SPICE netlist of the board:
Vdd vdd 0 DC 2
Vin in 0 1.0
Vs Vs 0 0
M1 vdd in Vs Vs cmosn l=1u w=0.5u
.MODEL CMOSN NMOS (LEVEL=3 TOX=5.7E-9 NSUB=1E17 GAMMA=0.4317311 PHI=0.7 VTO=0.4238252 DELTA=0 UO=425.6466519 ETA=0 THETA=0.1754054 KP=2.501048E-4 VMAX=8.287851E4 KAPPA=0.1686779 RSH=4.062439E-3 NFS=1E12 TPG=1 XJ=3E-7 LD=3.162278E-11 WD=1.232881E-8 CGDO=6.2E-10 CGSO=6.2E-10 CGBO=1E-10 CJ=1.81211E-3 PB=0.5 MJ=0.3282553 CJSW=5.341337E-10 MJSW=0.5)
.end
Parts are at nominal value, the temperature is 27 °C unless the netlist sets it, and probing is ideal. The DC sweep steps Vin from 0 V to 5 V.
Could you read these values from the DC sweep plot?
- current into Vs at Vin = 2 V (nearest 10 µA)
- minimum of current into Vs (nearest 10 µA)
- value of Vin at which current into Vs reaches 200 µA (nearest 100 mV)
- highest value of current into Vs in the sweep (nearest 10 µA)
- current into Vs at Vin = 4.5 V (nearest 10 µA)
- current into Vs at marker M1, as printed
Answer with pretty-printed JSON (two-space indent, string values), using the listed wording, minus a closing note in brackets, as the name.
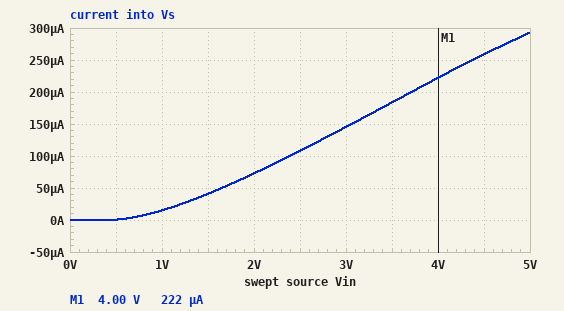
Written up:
{
  "current into Vs at Vin = 2 V": "70 µA",
  "minimum of current into Vs": "0 A",
  "value of Vin at which current into Vs reaches 200 µA": "3.7 V",
  "highest value of current into Vs in the sweep": "290 µA",
  "current into Vs at Vin = 4.5 V": "260 µA",
  "current into Vs at marker M1, as printed": "222 µA"
}
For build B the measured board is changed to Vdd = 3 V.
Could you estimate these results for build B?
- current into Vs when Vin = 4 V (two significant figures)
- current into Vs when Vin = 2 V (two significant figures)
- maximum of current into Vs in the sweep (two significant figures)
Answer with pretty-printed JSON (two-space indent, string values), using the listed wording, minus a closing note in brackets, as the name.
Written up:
{
  "current into Vs when Vin = 4 V": "230 µA",
  "current into Vs when Vin = 2 V": "74 µA",
  "maximum of current into Vs in the sweep": "310 µA"
}
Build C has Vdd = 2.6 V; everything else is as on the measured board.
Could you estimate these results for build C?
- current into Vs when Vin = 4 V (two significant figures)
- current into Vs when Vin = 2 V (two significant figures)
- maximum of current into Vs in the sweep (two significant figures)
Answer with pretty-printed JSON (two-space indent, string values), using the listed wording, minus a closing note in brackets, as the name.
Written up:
{
  "current into Vs when Vin = 4 V": "230 µA",
  "current into Vs when Vin = 2 V": "74 µA",
  "maximum of current into Vs in the sweep": "310 µA"
}
